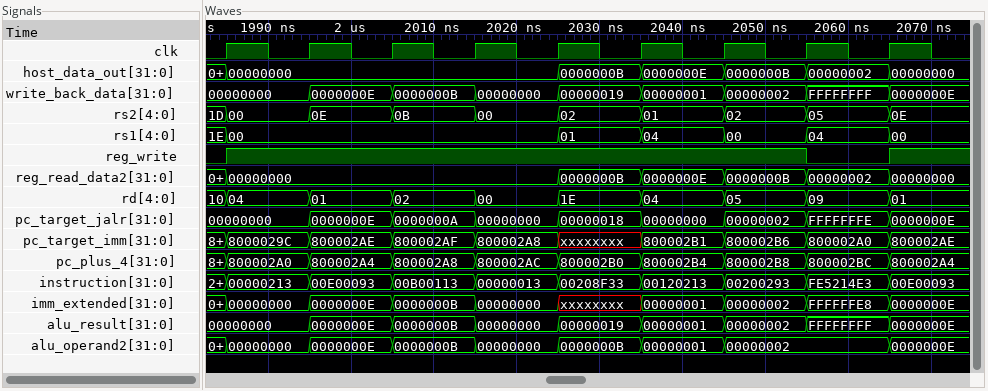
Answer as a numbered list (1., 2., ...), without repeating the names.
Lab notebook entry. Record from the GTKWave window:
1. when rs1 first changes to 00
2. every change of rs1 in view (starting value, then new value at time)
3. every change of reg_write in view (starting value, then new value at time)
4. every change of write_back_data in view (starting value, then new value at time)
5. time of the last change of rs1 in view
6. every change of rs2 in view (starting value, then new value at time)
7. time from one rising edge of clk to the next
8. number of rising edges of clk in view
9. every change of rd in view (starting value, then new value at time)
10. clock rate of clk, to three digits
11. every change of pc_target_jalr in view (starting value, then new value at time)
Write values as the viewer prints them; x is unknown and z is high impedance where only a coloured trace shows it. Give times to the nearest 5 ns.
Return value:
1. 1985 ns
2. 1E, 00 at 1985 ns, 01 at 2025 ns, 04 at 2035 ns, 00 at 2045 ns, 04 at 2055 ns, 00 at 2065 ns
3. 0, 1 at 1985 ns, 0 at 2055 ns, 1 at 2065 ns
4. 00000000, 0000000E at 1995 ns, 0000000B at 2005 ns, 00000000 at 2015 ns, 00000019 at 2025 ns, 00000001 at 2035 ns, 00000002 at 2045 ns, FFFFFFFF at 2055 ns, 0000000E at 2065 ns
5. 2065 ns
6. 1D, 00 at 1985 ns, 0E at 1995 ns, 0B at 2005 ns, 00 at 2015 ns, 02 at 2025 ns, 01 at 2035 ns, 02 at 2045 ns, 05 at 2055 ns, 0E at 2065 ns
7. 10 ns
8. 9
9. 10, 04 at 1985 ns, 01 at 1995 ns, 02 at 2005 ns, 00 at 2015 ns, 1E at 2025 ns, 04 at 2035 ns, 05 at 2045 ns, 09 at 2055 ns, 01 at 2065 ns
10. 100 MHz
11. 00000000, 0000000E at 1995 ns, 0000000A at 2005 ns, 00000000 at 2015 ns, 00000018 at 2025 ns, 00000000 at 2035 ns, 00000002 at 2045 ns, FFFFFFFE at 2055 ns, 0000000E at 2065 ns
